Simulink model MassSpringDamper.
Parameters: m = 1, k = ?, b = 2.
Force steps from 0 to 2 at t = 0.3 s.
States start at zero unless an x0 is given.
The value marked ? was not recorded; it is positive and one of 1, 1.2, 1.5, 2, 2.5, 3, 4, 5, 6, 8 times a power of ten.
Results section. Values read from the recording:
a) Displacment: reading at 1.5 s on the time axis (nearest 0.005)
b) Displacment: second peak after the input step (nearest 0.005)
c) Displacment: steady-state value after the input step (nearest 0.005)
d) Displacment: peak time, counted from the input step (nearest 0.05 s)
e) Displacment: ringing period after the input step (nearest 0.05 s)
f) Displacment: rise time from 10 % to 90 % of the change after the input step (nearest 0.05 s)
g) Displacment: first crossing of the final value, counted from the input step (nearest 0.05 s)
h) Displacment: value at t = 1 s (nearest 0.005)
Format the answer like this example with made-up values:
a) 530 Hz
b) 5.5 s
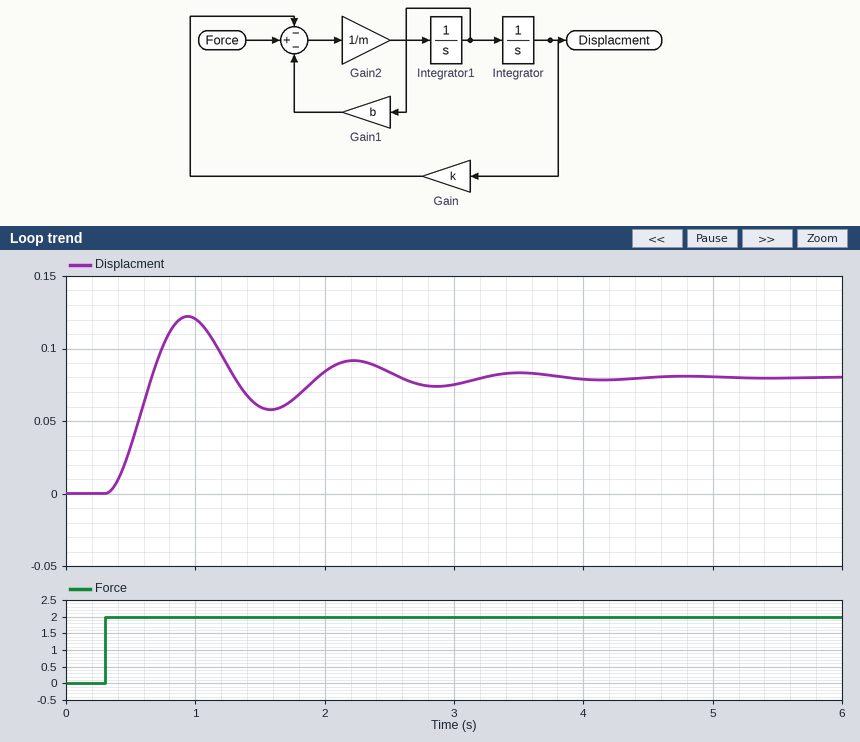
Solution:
a) 0.060
b) 0.090
c) 0.080
d) 0.65 s
e) 1.30 s
f) 0.25 s
g) 0.35 s
h) 0.120
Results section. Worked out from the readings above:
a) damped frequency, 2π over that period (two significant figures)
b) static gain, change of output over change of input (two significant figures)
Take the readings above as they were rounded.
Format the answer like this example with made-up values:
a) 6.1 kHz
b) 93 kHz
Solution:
a) 4.8 rad/s
b) 0.040
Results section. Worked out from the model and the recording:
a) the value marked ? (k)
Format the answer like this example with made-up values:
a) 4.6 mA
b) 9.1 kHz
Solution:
a) 25
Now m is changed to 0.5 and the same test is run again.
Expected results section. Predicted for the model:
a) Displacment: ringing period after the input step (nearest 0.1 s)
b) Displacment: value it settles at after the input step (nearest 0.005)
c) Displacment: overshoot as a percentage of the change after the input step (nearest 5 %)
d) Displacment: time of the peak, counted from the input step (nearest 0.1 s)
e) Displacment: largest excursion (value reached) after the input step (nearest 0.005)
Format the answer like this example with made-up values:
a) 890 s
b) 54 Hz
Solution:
a) 0.9 s
b) 0.080
c) 40 %
d) 0.5 s
e) 0.110
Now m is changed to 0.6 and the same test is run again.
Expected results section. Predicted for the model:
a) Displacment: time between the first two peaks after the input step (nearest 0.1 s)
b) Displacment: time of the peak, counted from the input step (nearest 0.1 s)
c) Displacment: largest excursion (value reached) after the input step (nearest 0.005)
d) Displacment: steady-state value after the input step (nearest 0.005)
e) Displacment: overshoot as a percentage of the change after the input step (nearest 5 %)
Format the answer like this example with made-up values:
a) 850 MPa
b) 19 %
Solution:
a) 1.0 s
b) 0.5 s
c) 0.115
d) 0.080
e) 45 %
